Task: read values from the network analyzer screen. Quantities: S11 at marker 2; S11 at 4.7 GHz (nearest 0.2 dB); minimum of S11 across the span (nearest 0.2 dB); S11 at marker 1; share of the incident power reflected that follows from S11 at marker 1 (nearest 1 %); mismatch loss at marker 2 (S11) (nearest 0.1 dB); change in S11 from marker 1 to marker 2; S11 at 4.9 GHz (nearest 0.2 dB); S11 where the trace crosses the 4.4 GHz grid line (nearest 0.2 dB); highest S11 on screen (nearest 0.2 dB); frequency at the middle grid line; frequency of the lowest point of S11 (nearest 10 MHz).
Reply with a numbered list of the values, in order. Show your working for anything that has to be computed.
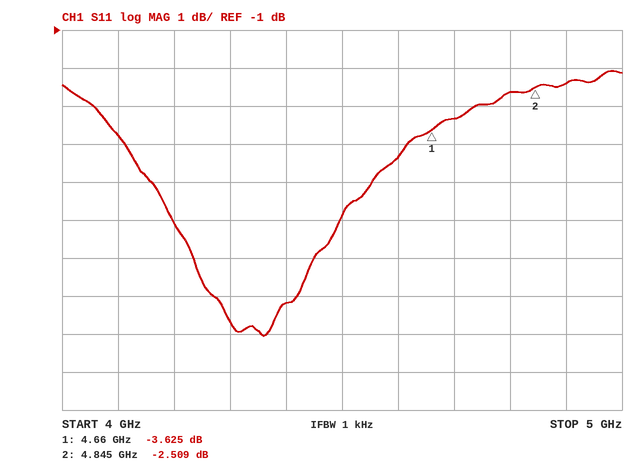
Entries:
1. -2.509 dB
2. -3.4 dB
3. -9.0 dB
4. -3.625 dB
5. 10^(-3.625/10) ≈ 43 %
6. −10 log10(1 − 10^(-2.509/10)) ≈ 3.6 dB
7. -2.509 − (-3.625) = 1.116 dB
8. -2.4 dB
9. -8.2 dB
10. -2.0 dB
11. 4.5 GHz
12. 4.36 GHz
